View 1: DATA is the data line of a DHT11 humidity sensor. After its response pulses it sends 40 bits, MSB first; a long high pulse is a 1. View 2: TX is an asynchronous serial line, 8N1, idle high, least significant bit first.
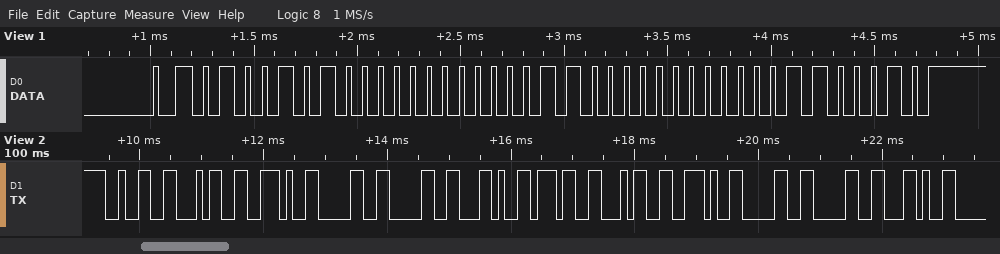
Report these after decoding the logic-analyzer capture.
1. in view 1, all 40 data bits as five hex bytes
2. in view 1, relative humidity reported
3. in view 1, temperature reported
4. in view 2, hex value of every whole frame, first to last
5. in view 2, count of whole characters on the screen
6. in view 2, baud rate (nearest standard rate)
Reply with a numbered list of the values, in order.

1. 4A 00 18 00 62
2. 74 %
3. 24.0 °C
4. 0x32 0x34 0x2E 0x30 0x30 0x2C 0x37 0x34 0x2E 0x30 0x30 0x2C
5. 12
6. 9600 baud
